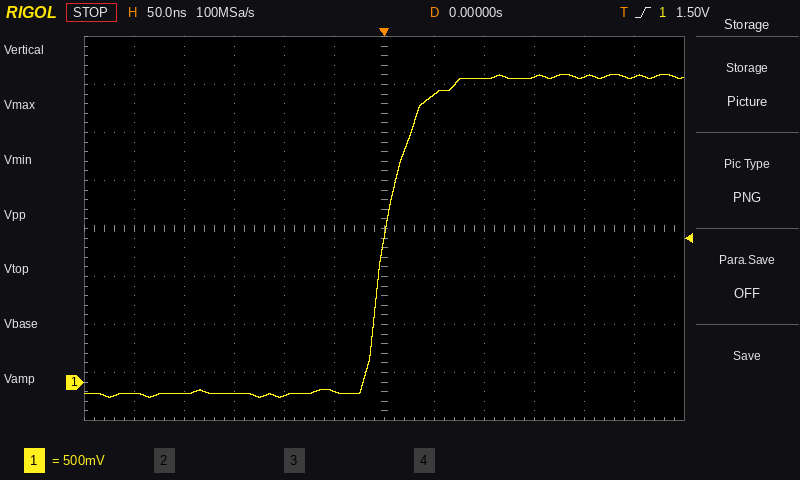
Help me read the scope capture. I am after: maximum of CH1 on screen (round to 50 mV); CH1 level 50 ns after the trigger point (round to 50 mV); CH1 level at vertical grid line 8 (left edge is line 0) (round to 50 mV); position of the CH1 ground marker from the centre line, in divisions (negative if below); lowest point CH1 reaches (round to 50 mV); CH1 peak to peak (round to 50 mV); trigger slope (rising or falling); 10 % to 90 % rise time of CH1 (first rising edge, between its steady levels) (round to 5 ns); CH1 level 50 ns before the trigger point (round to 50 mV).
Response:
3.20 V
3.00 V
3.15 V
-3.2 div
-150 mV
3.35 V
rising
50 ns
-100 mV
